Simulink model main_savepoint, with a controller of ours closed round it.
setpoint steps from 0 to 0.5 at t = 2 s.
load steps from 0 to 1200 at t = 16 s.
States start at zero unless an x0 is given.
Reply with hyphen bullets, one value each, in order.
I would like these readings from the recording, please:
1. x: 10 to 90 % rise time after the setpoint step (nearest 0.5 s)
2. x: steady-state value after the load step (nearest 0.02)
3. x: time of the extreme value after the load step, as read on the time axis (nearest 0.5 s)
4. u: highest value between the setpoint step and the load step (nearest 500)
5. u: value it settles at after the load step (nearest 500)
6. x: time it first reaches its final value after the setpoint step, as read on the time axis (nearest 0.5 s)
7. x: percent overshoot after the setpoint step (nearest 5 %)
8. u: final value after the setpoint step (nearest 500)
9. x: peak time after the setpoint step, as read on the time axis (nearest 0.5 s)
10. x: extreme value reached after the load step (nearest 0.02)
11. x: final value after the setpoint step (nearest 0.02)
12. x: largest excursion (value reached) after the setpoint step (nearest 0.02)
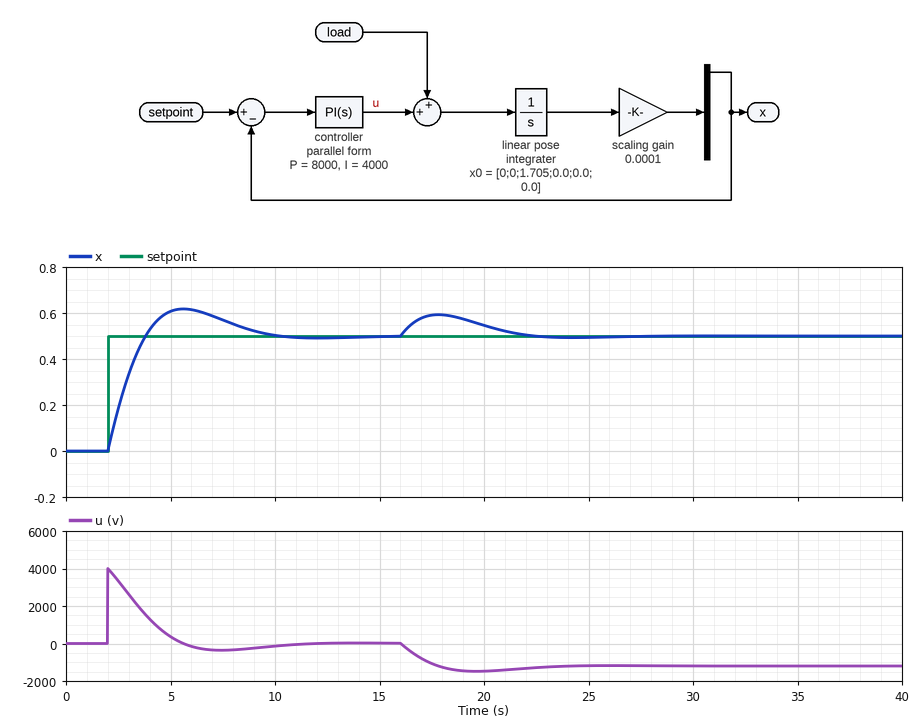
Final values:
- 1.5 s
- 0.50
- 18.0 s
- 4000
- -1000
- 4.0 s
- 25 %
- 0
- 5.5 s
- 0.60
- 0.50
- 0.62
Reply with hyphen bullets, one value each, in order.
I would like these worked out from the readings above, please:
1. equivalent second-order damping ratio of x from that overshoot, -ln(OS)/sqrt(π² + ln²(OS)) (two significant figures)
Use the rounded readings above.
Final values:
- 0.40
